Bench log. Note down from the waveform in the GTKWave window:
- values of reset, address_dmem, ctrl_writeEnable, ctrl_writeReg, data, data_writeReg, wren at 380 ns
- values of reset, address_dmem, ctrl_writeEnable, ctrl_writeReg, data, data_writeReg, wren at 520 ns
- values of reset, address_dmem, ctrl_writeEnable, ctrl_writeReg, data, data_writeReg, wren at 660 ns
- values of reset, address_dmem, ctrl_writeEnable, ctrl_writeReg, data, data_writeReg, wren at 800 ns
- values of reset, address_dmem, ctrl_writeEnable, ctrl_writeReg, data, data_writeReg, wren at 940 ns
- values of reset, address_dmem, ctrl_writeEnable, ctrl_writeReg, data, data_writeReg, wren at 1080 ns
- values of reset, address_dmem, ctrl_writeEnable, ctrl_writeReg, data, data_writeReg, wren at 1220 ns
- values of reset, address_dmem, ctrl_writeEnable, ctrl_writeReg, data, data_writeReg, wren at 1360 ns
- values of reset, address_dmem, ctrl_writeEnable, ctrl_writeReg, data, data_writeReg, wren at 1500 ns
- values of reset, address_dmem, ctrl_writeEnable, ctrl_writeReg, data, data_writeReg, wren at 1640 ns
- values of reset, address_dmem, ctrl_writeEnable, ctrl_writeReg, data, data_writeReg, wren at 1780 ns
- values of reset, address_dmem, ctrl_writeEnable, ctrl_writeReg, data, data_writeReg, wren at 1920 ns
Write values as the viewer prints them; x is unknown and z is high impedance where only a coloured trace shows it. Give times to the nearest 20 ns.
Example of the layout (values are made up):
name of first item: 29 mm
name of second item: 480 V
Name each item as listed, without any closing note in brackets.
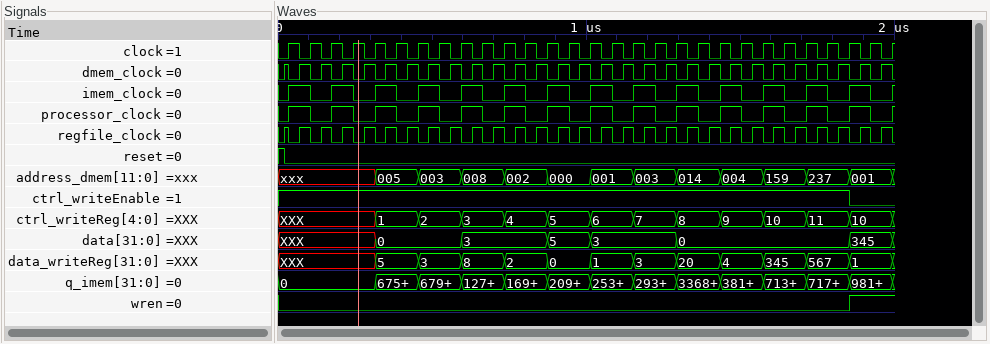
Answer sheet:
values of reset, address_dmem, ctrl_writeEnable, ctrl_writeReg, data, data_writeReg, wren at 380 ns: reset=0, address_dmem=005, ctrl_writeEnable=1, ctrl_writeReg=1, data=0, data_writeReg=5, wren=0
values of reset, address_dmem, ctrl_writeEnable, ctrl_writeReg, data, data_writeReg, wren at 520 ns: reset=0, address_dmem=003, ctrl_writeEnable=1, ctrl_writeReg=2, data=0, data_writeReg=3, wren=0
values of reset, address_dmem, ctrl_writeEnable, ctrl_writeReg, data, data_writeReg, wren at 660 ns: reset=0, address_dmem=008, ctrl_writeEnable=1, ctrl_writeReg=3, data=3, data_writeReg=8, wren=0
values of reset, address_dmem, ctrl_writeEnable, ctrl_writeReg, data, data_writeReg, wren at 800 ns: reset=0, address_dmem=002, ctrl_writeEnable=1, ctrl_writeReg=4, data=3, data_writeReg=2, wren=0
values of reset, address_dmem, ctrl_writeEnable, ctrl_writeReg, data, data_writeReg, wren at 940 ns: reset=0, address_dmem=000, ctrl_writeEnable=1, ctrl_writeReg=5, data=5, data_writeReg=0, wren=0
values of reset, address_dmem, ctrl_writeEnable, ctrl_writeReg, data, data_writeReg, wren at 1080 ns: reset=0, address_dmem=001, ctrl_writeEnable=1, ctrl_writeReg=6, data=3, data_writeReg=1, wren=0
values of reset, address_dmem, ctrl_writeEnable, ctrl_writeReg, data, data_writeReg, wren at 1220 ns: reset=0, address_dmem=003, ctrl_writeEnable=1, ctrl_writeReg=7, data=3, data_writeReg=3, wren=0
values of reset, address_dmem, ctrl_writeEnable, ctrl_writeReg, data, data_writeReg, wren at 1360 ns: reset=0, address_dmem=014, ctrl_writeEnable=1, ctrl_writeReg=8, data=0, data_writeReg=20, wren=0
values of reset, address_dmem, ctrl_writeEnable, ctrl_writeReg, data, data_writeReg, wren at 1500 ns: reset=0, address_dmem=004, ctrl_writeEnable=1, ctrl_writeReg=9, data=0, data_writeReg=4, wren=0
values of reset, address_dmem, ctrl_writeEnable, ctrl_writeReg, data, data_writeReg, wren at 1640 ns: reset=0, address_dmem=159, ctrl_writeEnable=1, ctrl_writeReg=10, data=0, data_writeReg=345, wren=0
values of reset, address_dmem, ctrl_writeEnable, ctrl_writeReg, data, data_writeReg, wren at 1780 ns: reset=0, address_dmem=237, ctrl_writeEnable=1, ctrl_writeReg=11, data=0, data_writeReg=567, wren=0
values of reset, address_dmem, ctrl_writeEnable, ctrl_writeReg, data, data_writeReg, wren at 1920 ns: reset=0, address_dmem=001, ctrl_writeEnable=0, ctrl_writeReg=10, data=345, data_writeReg=1, wren=1
